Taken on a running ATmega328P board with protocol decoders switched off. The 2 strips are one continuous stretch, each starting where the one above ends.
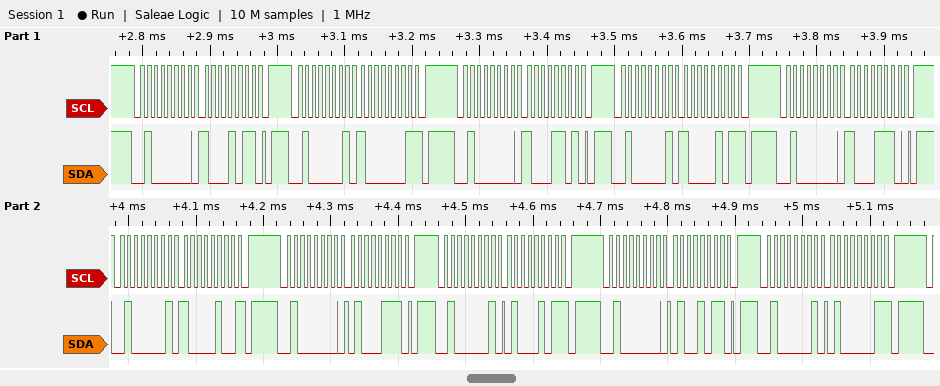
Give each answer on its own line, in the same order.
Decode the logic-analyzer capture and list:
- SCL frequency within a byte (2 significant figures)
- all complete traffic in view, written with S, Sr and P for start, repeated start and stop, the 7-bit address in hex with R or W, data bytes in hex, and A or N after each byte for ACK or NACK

100 kHz
S 20W A 8B A P S 20R A 81 N P S 20W A 8D A P S 20R A 85 N P S 20W A 8E A P S 20R A 84 N P S 20W A 47 A P S 20R A 45 N P S 20W A 4B A P S 20R A 41 N P
